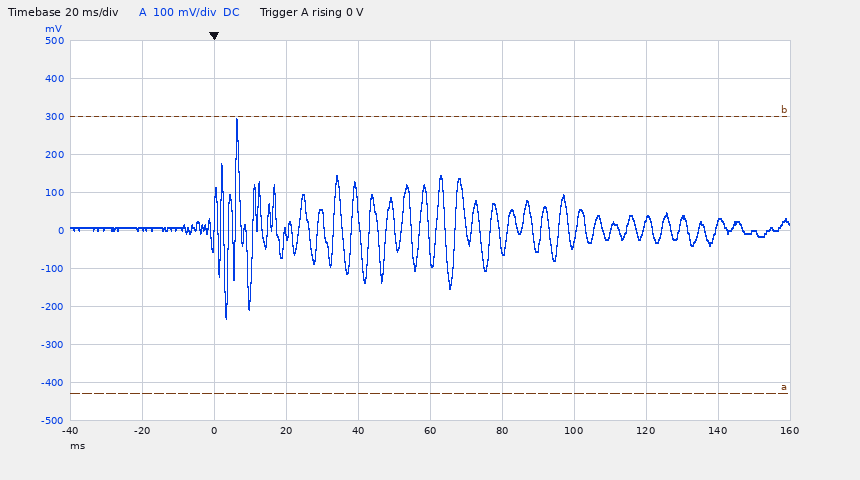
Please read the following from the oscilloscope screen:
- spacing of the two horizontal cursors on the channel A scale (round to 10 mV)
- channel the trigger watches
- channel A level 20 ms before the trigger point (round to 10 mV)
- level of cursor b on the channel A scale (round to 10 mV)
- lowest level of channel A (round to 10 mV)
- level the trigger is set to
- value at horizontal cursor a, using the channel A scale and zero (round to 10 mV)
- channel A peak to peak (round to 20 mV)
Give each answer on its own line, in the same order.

730 mV
channel A
0 mV
300 mV
-230 mV
0 V
-430 mV
520 mV
